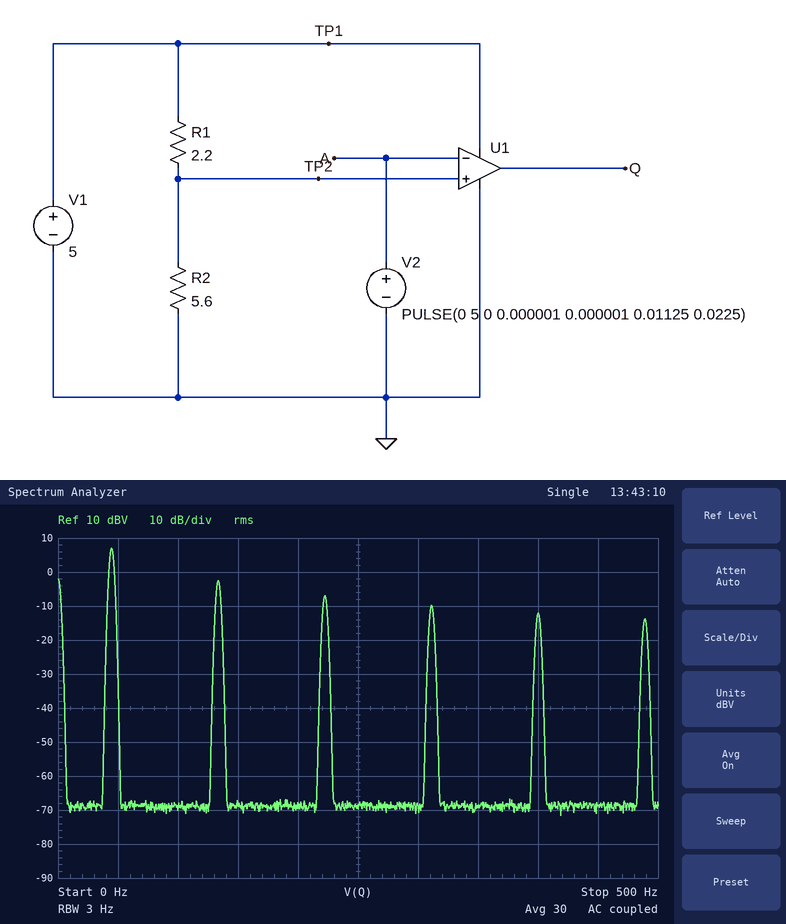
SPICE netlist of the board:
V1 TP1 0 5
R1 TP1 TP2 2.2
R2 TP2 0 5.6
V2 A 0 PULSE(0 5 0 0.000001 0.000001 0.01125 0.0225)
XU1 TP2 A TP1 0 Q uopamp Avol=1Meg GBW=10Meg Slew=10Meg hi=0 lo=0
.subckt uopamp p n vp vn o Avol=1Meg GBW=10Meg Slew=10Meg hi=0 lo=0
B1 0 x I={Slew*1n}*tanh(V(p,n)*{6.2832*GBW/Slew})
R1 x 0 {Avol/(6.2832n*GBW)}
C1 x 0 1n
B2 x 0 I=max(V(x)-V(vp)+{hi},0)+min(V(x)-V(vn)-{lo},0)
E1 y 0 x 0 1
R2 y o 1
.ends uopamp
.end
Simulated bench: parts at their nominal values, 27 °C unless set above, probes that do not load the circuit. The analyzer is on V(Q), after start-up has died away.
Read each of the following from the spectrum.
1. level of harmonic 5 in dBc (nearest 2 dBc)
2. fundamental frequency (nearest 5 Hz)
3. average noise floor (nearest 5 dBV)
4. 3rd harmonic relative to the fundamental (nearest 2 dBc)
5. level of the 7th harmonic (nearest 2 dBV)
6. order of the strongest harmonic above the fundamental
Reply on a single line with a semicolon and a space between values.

-14 dBc; 45 Hz; -70 dBV; -10 dBc; -10 dBV; 3
